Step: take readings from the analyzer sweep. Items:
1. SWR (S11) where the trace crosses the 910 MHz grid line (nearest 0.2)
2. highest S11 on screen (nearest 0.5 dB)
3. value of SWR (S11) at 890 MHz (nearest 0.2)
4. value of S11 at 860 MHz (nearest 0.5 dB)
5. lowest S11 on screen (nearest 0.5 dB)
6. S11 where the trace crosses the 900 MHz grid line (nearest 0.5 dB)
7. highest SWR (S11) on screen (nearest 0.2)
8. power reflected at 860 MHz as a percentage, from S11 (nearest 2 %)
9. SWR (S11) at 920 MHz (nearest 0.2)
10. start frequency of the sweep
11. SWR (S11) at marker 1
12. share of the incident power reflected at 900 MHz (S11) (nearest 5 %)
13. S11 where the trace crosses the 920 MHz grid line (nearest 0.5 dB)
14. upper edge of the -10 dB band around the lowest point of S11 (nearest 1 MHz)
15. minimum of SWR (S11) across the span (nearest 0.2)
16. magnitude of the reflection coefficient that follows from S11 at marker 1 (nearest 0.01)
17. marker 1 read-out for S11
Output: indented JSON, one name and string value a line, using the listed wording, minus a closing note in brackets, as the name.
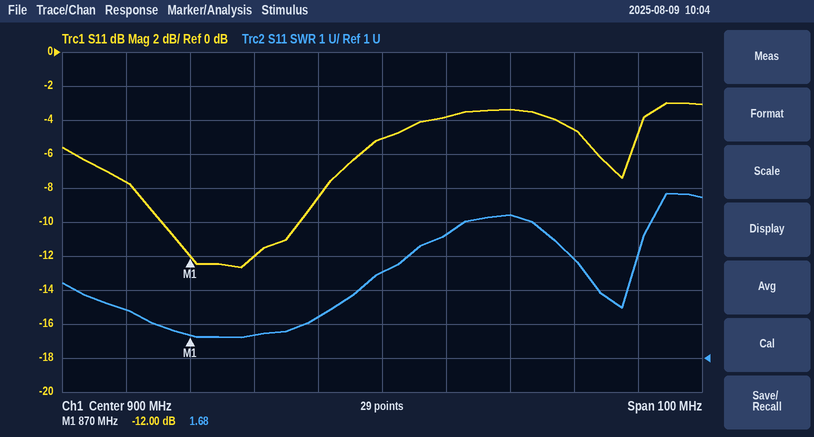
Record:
{
  "SWR (S11) where the trace crosses the 910 MHz grid line": "4.6",
  "highest S11 on screen": "-3.0 dB",
  "value of SWR (S11) at 890 MHz": "2.2",
  "value of S11 at 860 MHz": "-7.5 dB",
  "lowest S11 on screen": "-12.5 dB",
  "S11 where the trace crosses the 900 MHz grid line": "-5.0 dB",
  "highest SWR (S11) on screen": "5.8",
  "power reflected at 860 MHz as a percentage, from S11": "18 %",
  "SWR (S11) at 920 MHz": "5.2",
  "start frequency of the sweep": "850 MHz",
  "SWR (S11) at marker 1": "1.68",
  "share of the incident power reflected at 900 MHz (S11)": "30 %",
  "S11 where the trace crosses the 920 MHz grid line": "-3.5 dB",
  "upper edge of the -10 dB band around the lowest point of S11": "887 MHz",
  "minimum of SWR (S11) across the span": "1.6",
  "magnitude of the reflection coefficient that follows from S11 at marker 1": "0.25",
  "marker 1 read-out for S11": "-12.00 dB"
}
